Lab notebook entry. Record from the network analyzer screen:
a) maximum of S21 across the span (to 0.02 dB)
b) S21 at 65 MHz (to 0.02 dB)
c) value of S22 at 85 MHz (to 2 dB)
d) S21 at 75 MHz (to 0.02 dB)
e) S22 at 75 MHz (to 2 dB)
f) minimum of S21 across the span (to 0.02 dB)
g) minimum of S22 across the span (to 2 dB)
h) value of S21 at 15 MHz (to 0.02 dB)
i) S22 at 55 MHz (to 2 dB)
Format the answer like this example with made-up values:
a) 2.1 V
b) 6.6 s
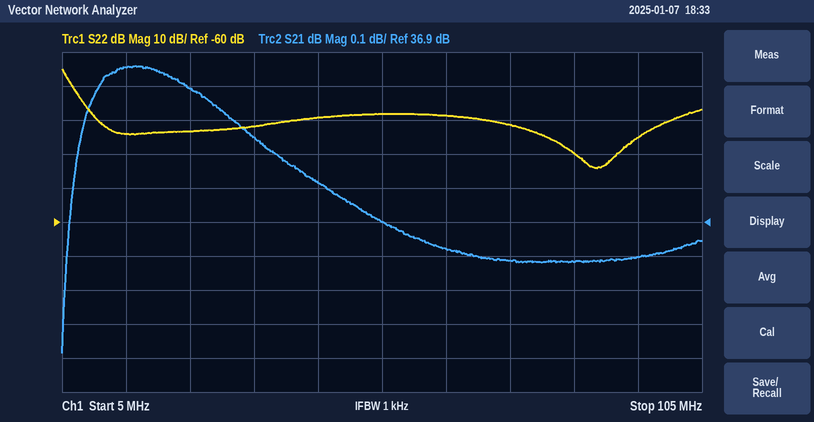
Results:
a) 37.36 dB
b) 36.82 dB
c) -40 dB
d) 36.78 dB
e) -32 dB
f) 36.52 dB
g) -44 dB
h) 37.36 dB
i) -28 dB
